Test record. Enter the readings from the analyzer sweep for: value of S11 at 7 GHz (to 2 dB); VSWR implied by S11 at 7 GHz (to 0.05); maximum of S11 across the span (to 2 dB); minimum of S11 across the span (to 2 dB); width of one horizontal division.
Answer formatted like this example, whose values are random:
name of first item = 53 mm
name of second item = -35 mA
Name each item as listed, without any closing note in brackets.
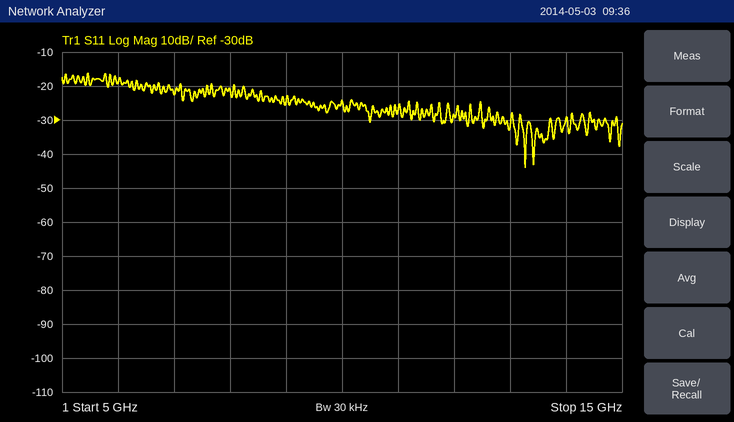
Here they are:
value of S11 at 7 GHz = -22 dB
VSWR implied by S11 at 7 GHz = 1.15
maximum of S11 across the span = -16 dB
minimum of S11 across the span = -44 dB
width of one horizontal division = 1 GHz
